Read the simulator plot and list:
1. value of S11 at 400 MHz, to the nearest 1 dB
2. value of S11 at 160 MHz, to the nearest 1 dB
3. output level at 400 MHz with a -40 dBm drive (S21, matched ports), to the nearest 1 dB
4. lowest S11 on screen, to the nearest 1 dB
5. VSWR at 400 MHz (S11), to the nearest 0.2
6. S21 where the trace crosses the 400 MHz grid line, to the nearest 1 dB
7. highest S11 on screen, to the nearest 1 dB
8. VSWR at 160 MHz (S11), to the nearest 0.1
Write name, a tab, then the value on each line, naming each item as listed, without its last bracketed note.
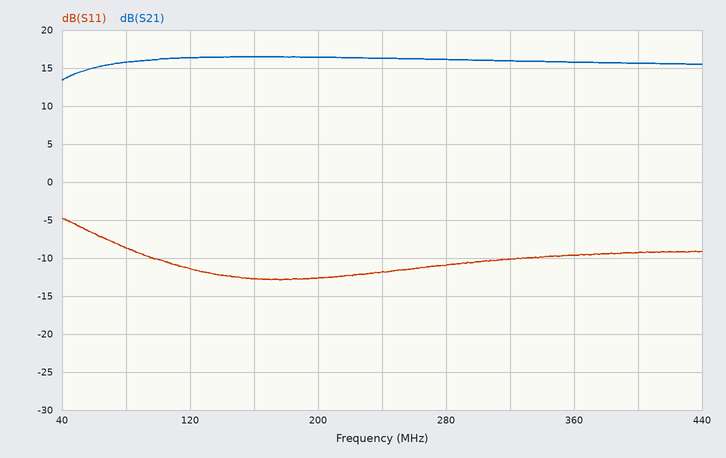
value of S11 at 400 MHz, to the nearest 1 dB	-9 dB
value of S11 at 160 MHz, to the nearest 1 dB	-13 dB
output level at 400 MHz with a -40 dBm drive (S21, matched ports), to the nearest 1 dB	-24 dBm
lowest S11 on screen, to the nearest 1 dB	-13 dB
VSWR at 400 MHz (S11), to the nearest 0.2	2.0
S21 where the trace crosses the 400 MHz grid line, to the nearest 1 dB	16 dB
highest S11 on screen, to the nearest 1 dB	-5 dB
VSWR at 160 MHz (S11), to the nearest 0.1	1.6
